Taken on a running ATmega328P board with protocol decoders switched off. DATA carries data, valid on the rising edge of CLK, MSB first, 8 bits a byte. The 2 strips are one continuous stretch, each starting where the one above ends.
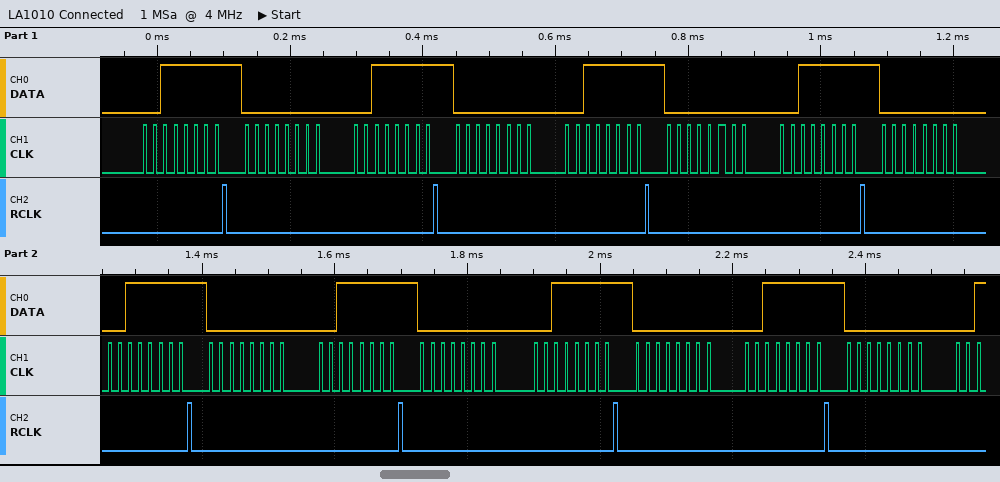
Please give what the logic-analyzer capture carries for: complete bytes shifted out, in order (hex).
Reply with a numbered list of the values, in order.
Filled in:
1. 0x3F 0x00 0x3F 0x00 0x3F 0x00 0x3F 0x00 0x3F 0x00 0x3F 0x00 0x3F 0x00 0x3F 0x00
